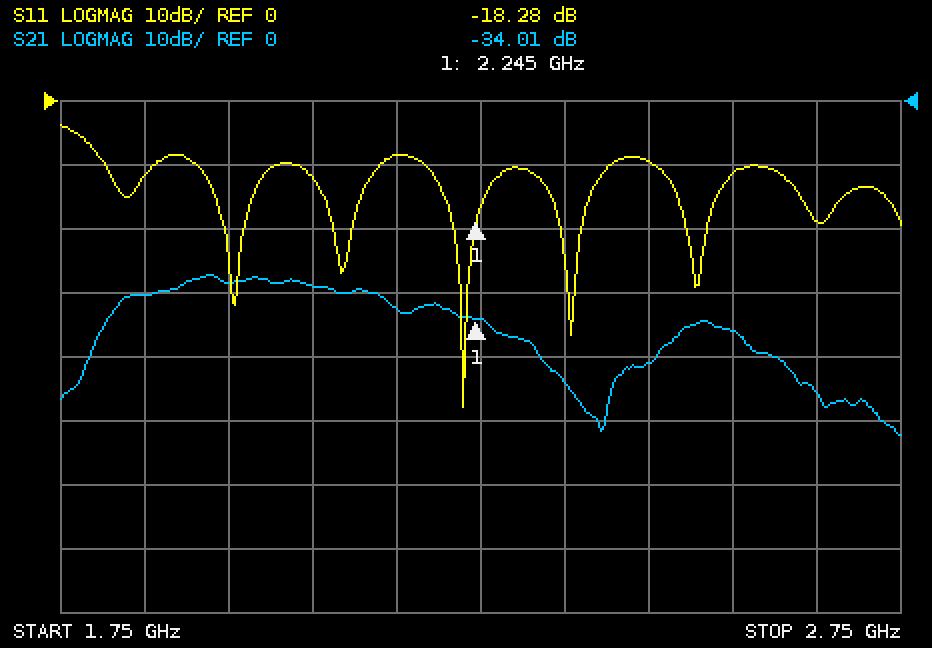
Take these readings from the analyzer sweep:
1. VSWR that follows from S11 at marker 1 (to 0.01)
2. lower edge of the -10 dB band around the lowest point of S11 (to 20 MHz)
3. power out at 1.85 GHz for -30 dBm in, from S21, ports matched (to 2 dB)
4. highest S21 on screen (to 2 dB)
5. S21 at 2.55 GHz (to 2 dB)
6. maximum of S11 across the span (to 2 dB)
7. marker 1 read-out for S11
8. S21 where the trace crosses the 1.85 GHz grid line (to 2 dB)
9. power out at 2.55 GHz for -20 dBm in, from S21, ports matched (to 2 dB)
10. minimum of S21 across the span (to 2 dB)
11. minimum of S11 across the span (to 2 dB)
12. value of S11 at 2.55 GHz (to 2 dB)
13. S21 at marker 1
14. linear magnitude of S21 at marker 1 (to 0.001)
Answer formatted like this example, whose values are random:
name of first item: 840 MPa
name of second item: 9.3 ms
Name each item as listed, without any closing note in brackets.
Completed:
VSWR that follows from S11 at marker 1: 1.28
lower edge of the -10 dB band around the lowest point of S11: 2.18 GHz
power out at 1.85 GHz for -30 dBm in, from S21, ports matched: -60 dBm
highest S21 on screen: -28 dB
S21 at 2.55 GHz: -36 dB
maximum of S11 across the span: -4 dB
marker 1 read-out for S11: -18.28 dB
S21 where the trace crosses the 1.85 GHz grid line: -30 dB
power out at 2.55 GHz for -20 dBm in, from S21, ports matched: -56 dBm
minimum of S21 across the span: -52 dB
minimum of S11 across the span: -48 dB
value of S11 at 2.55 GHz: -12 dB
S21 at marker 1: -34.01 dB
linear magnitude of S21 at marker 1: 0.020
